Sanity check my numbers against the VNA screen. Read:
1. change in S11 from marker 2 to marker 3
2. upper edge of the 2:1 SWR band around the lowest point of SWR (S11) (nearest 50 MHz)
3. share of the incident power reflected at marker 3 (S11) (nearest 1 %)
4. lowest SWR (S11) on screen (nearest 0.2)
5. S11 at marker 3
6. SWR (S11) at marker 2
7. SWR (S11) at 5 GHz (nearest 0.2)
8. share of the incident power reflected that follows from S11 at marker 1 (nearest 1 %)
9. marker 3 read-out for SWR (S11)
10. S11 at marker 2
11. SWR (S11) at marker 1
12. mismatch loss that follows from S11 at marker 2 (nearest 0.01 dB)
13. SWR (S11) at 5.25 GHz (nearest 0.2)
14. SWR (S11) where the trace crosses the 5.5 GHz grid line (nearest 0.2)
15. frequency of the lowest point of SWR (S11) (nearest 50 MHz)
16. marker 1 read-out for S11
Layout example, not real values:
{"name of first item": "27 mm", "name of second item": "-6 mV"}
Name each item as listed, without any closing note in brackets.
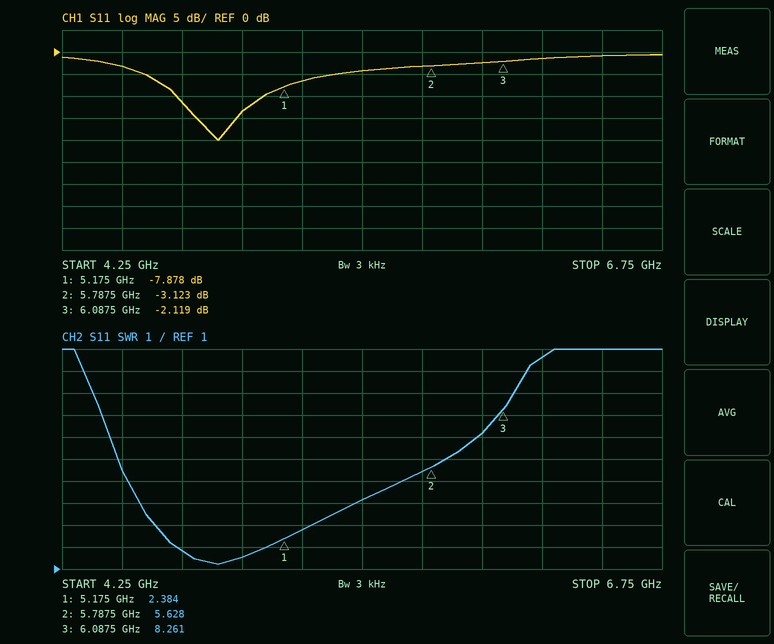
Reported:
{"change in S11 from marker 2 to marker 3": "1.004 dB", "upper edge of the 2:1 SWR band around the lowest point of SWR (S11)": "5.10 GHz", "share of the incident power reflected at marker 3 (S11)": "61 %", "lowest SWR (S11) on screen": "1.2", "S11 at marker 3": "-2.119 dB", "SWR (S11) at marker 2": "5.628", "SWR (S11) at 5 GHz": "1.6", "share of the incident power reflected that follows from S11 at marker 1": "16 %", "marker 3 read-out for SWR": "8.261", "S11 at marker 2": "-3.123 dB", "SWR (S11) at marker 1": "2.384", "mismatch loss that follows from S11 at marker 2": "2.90 dB", "SWR (S11) at 5.25 GHz": "2.8", "SWR (S11) where the trace crosses the 5.5 GHz grid line": "4.2", "frequency of the lowest point of SWR (S11)": "4.90 GHz", "marker 1 read-out for S11": "-7.878 dB"}
